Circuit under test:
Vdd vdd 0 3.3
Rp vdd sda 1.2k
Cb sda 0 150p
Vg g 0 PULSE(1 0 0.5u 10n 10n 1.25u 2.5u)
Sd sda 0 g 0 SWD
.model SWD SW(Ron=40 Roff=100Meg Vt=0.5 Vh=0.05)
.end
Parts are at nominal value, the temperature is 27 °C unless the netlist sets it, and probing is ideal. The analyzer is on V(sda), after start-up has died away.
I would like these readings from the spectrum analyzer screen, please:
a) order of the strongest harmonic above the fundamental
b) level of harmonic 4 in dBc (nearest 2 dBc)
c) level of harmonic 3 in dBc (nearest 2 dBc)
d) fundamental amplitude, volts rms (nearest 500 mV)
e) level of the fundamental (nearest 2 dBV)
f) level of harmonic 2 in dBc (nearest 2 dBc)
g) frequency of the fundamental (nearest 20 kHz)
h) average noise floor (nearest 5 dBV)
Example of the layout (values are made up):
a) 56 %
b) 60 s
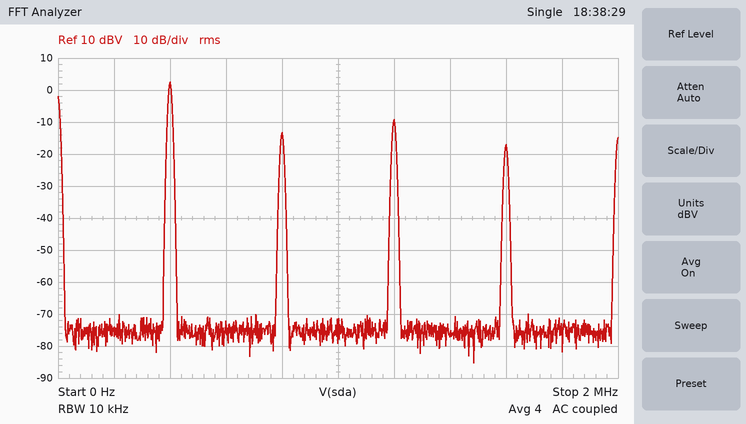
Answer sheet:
a) 3
b) -20 dBc
c) -12 dBc
d) 1.5 V
e) 2 dBV
f) -16 dBc
g) 400 kHz
h) -75 dBV
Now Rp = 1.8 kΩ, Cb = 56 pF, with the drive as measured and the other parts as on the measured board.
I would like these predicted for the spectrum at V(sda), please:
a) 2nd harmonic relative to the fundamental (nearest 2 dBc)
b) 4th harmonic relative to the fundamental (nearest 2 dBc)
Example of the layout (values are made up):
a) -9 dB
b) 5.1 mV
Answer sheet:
a) -20 dBc
b) -22 dBc
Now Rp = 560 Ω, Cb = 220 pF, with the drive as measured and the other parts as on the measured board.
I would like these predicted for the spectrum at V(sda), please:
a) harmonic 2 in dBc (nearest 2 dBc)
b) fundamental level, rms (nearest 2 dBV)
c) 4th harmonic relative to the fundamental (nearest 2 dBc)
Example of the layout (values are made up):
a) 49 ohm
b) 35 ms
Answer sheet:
a) -18 dBc
b) 2 dBV
c) -22 dBc
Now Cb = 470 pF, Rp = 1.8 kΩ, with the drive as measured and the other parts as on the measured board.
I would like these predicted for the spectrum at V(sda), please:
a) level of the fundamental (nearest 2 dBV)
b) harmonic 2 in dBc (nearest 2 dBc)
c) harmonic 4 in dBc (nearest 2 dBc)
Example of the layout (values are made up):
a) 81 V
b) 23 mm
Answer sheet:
a) -2 dBV
b) -10 dBc
c) -16 dBc
